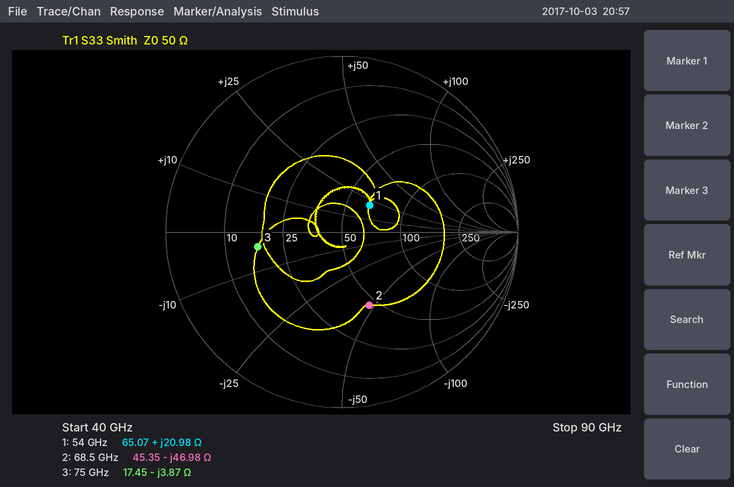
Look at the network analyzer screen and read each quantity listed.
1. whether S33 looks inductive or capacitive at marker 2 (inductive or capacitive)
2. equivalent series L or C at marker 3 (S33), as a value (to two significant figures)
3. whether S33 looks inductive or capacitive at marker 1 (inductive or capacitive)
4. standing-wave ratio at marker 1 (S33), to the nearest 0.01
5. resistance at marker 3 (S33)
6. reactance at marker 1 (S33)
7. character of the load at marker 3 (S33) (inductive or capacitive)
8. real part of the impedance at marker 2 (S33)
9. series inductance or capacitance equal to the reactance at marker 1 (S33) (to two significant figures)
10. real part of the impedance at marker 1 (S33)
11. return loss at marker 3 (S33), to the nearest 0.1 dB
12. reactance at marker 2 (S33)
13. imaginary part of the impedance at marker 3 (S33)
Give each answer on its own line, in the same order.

capacitive
550 fF
inductive
1.57
17.45 Ω
+20.98 Ω
capacitive
45.35 Ω
62 pH
65.07 Ω
6.3 dB
-46.98 Ω
-3.87 Ω
